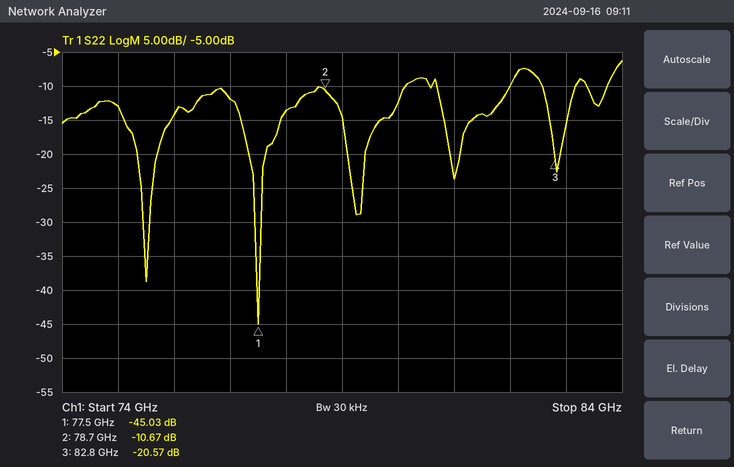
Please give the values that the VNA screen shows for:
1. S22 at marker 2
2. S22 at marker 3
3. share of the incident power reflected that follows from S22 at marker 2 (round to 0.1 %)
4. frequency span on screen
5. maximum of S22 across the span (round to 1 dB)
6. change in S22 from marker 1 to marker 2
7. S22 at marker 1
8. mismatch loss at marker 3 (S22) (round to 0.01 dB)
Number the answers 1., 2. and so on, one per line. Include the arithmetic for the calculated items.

1. -10.67 dB
2. -20.57 dB
3. 10^(-10.67/10) ≈ 8.6 %
4. 10 GHz
5. -6 dB
6. -10.67 − (-45.03) = 34.36 dB
7. -45.03 dB
8. −10 log10(1 − 10^(-20.57/10)) ≈ 0.04 dB
